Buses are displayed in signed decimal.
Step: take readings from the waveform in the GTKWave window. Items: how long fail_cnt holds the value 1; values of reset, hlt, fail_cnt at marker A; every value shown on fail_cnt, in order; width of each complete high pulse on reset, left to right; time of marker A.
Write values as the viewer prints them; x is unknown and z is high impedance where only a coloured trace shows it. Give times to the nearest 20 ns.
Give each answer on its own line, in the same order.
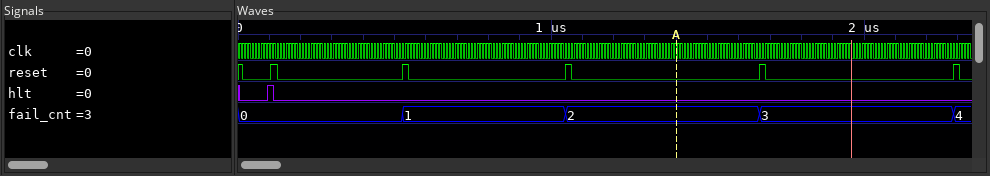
520 ns
reset=0, hlt=0, fail_cnt=2
0, 1, 2, 3, 4
20 ns, 20 ns, 20 ns, 20 ns, 20 ns
1400 ns
